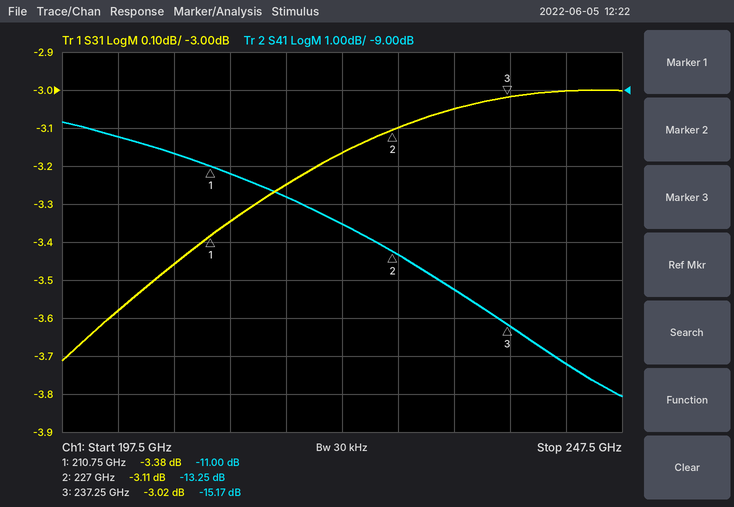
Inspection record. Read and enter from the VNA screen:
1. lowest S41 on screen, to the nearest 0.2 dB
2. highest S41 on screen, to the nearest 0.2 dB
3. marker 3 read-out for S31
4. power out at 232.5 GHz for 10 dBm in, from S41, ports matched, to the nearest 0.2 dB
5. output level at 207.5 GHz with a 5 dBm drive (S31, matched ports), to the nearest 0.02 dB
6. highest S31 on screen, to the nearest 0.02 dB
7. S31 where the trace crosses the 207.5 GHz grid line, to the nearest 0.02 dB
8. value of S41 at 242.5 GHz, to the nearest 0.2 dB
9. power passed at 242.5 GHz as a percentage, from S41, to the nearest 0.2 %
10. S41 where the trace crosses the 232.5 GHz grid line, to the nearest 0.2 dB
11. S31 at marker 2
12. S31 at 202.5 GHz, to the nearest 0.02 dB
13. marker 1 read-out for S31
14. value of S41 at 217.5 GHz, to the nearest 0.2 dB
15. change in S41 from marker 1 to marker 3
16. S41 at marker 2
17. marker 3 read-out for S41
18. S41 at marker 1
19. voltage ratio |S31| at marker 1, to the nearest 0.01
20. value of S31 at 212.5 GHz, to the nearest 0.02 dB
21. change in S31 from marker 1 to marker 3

-17.0 dB
-9.8 dB
-3.02 dB
-4.2 dBm
1.54 dBm
-3.00 dB
-3.46 dB
-16.2 dB
2.4 %
-14.2 dB
-3.11 dB
-3.58 dB
-3.38 dB
-11.8 dB
-4.17 dB
-13.25 dB
-15.17 dB
-11.00 dB
0.68
-3.34 dB
0.36 dB
